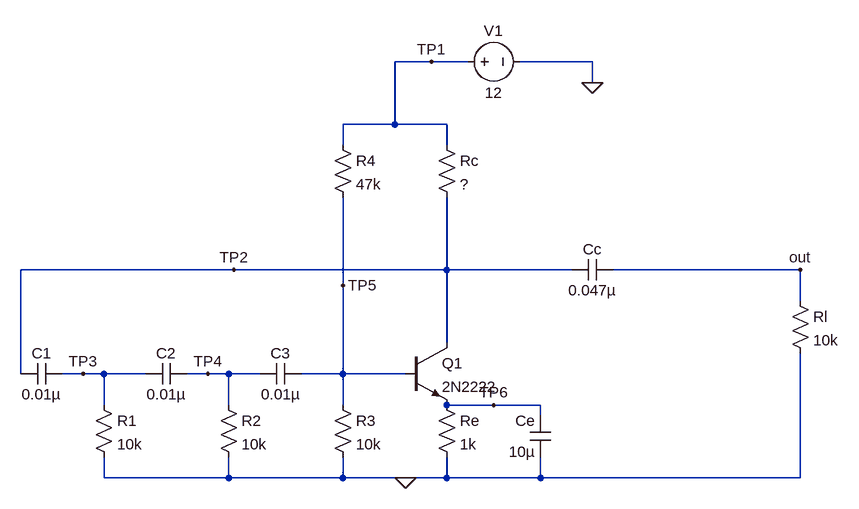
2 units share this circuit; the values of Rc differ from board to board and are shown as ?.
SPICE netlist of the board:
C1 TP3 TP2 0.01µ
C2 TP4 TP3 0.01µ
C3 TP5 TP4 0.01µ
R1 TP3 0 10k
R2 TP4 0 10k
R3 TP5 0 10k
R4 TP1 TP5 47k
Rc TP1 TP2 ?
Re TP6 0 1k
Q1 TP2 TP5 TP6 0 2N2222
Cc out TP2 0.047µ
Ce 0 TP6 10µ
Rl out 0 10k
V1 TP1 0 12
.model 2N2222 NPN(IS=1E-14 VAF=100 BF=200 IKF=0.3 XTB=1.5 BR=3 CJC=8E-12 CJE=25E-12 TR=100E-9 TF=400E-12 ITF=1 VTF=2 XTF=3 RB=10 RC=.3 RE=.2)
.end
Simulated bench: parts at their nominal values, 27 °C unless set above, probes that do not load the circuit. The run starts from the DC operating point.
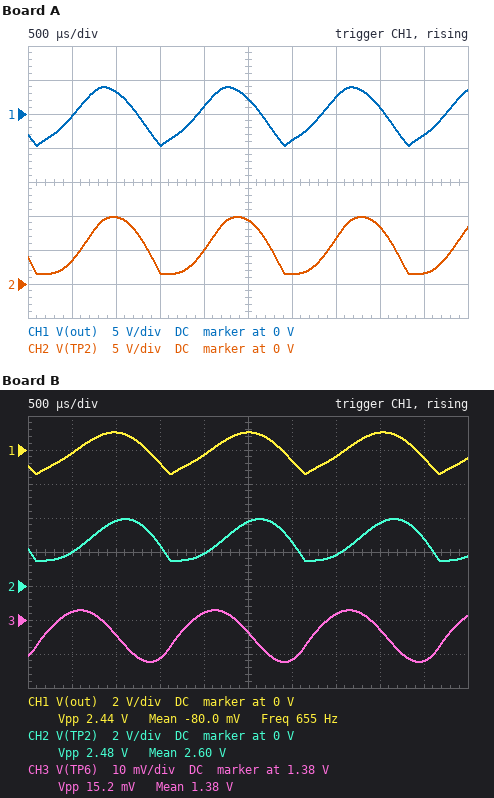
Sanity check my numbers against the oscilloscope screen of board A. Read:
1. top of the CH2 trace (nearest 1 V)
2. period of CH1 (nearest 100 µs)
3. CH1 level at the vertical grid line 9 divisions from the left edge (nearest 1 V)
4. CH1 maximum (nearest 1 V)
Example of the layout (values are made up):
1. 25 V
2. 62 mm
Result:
1. 10 V
2. 1.4 ms
3. -3 V
4. 4 V
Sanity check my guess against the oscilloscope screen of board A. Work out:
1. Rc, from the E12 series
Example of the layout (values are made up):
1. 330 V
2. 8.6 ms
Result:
1. 4.7 kΩ
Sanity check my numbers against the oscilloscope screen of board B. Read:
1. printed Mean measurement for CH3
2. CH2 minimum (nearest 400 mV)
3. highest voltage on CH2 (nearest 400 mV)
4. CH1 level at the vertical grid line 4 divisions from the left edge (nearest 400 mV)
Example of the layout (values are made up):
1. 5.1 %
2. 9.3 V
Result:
1. 1.38 V
2. 1.6 V
3. 4.0 V
4. -400 mV
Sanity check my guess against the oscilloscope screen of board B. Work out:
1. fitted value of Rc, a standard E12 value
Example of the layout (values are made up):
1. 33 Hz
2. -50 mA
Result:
1. 6.8 kΩ
